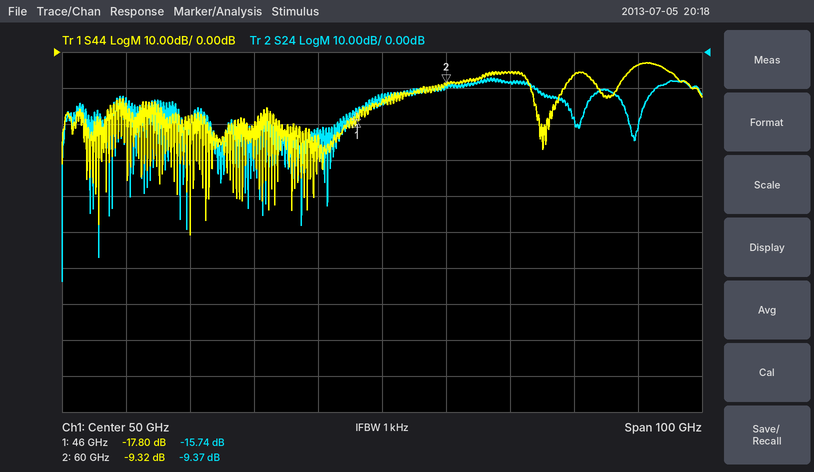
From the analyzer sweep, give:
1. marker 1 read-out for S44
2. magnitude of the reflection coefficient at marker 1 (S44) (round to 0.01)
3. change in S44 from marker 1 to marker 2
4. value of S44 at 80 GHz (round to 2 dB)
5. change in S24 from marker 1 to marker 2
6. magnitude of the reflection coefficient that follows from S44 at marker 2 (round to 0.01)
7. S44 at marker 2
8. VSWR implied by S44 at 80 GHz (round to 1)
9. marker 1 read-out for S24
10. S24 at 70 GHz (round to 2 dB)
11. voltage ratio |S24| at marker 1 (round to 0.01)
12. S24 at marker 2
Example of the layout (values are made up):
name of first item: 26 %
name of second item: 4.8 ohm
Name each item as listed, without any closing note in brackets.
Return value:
marker 1 read-out for S44: -17.80 dB
magnitude of the reflection coefficient at marker 1 (S44): 0.13
change in S44 from marker 1 to marker 2: 8.48 dB
value of S44 at 80 GHz: -6 dB
change in S24 from marker 1 to marker 2: 6.37 dB
magnitude of the reflection coefficient that follows from S44 at marker 2: 0.34
S44 at marker 2: -9.32 dB
VSWR implied by S44 at 80 GHz: 3
marker 1 read-out for S24: -15.74 dB
S24 at 70 GHz: -8 dB
voltage ratio |S24| at marker 1: 0.16
S24 at marker 2: -9.37 dB
